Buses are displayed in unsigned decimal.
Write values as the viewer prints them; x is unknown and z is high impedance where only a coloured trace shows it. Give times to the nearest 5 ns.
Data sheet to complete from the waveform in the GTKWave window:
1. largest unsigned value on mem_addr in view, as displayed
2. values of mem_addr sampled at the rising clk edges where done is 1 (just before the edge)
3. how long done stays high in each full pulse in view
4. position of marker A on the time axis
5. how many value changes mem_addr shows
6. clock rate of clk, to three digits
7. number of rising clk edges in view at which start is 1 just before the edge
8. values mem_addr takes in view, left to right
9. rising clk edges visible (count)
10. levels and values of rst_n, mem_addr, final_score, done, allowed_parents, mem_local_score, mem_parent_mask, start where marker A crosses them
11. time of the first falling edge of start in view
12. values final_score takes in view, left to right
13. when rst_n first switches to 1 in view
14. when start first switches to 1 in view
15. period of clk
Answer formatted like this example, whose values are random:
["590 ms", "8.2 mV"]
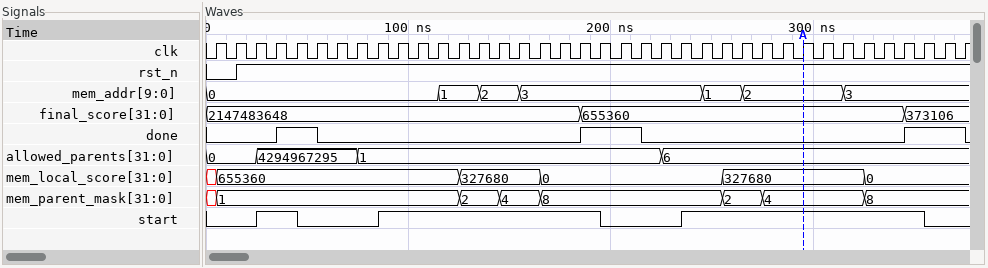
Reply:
["3", "0, 0, 3, 3, 3, 3, 3, 3", "20 ns, 30 ns, 30 ns", "295 ns", "6", "100 MHz", "25", "0, 1, 2, 3, 1, 2, 3", "38", "rst_n=1, mem_addr=2, final_score=655360, done=0, allowed_parents=6, mem_local_score=327680, mem_parent_mask=4, start=1", "45 ns", "2147483648, 655360, 373106", "15 ns", "25 ns", "10 ns"]
